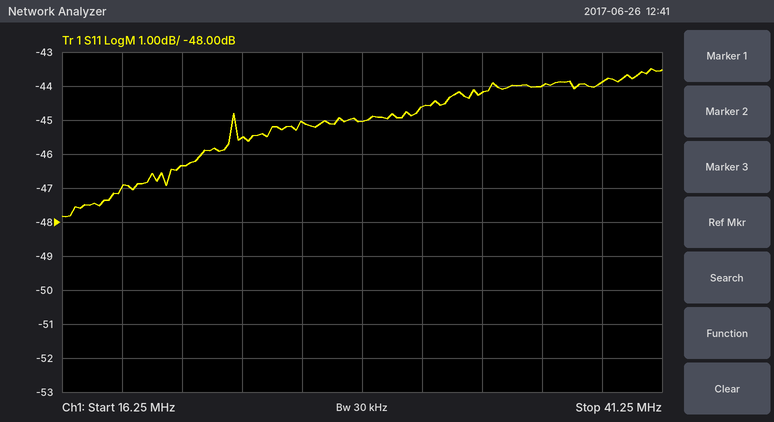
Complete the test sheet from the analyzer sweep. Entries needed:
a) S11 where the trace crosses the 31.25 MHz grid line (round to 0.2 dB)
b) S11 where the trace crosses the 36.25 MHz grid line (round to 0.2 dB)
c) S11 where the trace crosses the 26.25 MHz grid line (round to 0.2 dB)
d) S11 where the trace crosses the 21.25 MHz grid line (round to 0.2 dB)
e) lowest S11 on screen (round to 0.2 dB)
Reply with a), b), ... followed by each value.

a) -44.6 dB
b) -44.0 dB
c) -45.0 dB
d) -46.4 dB
e) -47.8 dB
